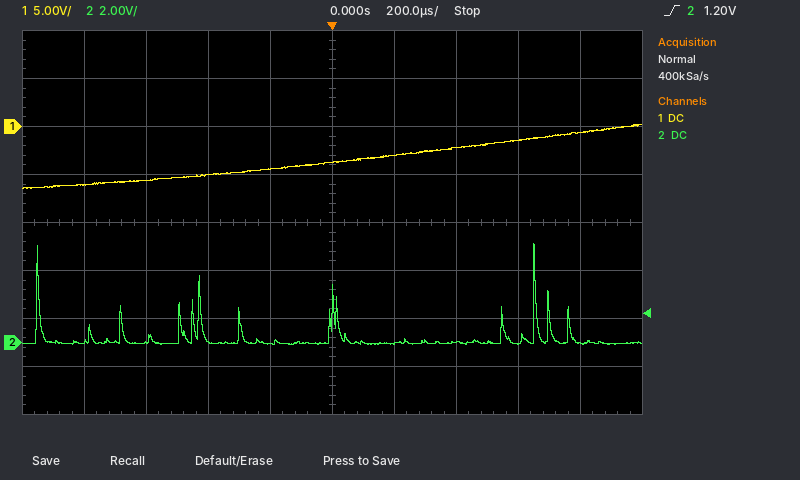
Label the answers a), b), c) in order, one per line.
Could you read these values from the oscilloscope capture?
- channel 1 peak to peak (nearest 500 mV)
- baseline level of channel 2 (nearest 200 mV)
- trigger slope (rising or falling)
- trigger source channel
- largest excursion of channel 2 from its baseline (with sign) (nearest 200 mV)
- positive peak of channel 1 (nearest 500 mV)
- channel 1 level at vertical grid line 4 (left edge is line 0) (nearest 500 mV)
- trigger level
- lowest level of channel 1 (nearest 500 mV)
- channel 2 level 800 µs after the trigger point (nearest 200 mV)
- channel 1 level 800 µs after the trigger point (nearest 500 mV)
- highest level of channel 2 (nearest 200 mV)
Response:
a) 6.5 V
b) 0.0 V
c) rising
d) channel 2
e) +4.2 V
f) 0.0 V
g) -4.5 V
h) 1.20 V
i) -6.5 V
j) 0.0 V
k) -500 mV
l) 4.2 V
